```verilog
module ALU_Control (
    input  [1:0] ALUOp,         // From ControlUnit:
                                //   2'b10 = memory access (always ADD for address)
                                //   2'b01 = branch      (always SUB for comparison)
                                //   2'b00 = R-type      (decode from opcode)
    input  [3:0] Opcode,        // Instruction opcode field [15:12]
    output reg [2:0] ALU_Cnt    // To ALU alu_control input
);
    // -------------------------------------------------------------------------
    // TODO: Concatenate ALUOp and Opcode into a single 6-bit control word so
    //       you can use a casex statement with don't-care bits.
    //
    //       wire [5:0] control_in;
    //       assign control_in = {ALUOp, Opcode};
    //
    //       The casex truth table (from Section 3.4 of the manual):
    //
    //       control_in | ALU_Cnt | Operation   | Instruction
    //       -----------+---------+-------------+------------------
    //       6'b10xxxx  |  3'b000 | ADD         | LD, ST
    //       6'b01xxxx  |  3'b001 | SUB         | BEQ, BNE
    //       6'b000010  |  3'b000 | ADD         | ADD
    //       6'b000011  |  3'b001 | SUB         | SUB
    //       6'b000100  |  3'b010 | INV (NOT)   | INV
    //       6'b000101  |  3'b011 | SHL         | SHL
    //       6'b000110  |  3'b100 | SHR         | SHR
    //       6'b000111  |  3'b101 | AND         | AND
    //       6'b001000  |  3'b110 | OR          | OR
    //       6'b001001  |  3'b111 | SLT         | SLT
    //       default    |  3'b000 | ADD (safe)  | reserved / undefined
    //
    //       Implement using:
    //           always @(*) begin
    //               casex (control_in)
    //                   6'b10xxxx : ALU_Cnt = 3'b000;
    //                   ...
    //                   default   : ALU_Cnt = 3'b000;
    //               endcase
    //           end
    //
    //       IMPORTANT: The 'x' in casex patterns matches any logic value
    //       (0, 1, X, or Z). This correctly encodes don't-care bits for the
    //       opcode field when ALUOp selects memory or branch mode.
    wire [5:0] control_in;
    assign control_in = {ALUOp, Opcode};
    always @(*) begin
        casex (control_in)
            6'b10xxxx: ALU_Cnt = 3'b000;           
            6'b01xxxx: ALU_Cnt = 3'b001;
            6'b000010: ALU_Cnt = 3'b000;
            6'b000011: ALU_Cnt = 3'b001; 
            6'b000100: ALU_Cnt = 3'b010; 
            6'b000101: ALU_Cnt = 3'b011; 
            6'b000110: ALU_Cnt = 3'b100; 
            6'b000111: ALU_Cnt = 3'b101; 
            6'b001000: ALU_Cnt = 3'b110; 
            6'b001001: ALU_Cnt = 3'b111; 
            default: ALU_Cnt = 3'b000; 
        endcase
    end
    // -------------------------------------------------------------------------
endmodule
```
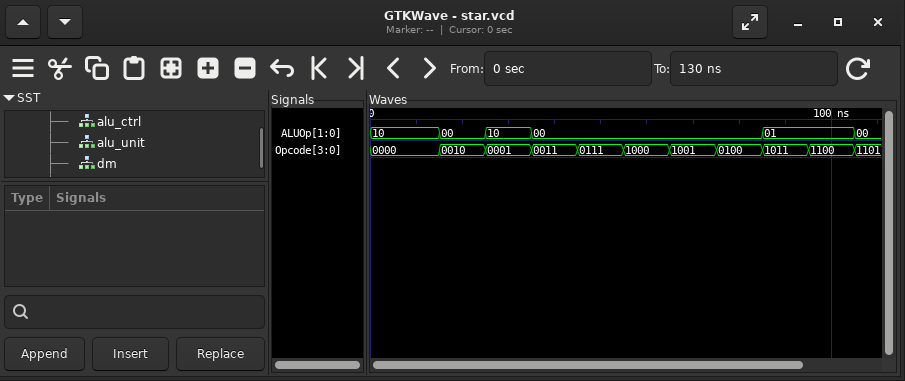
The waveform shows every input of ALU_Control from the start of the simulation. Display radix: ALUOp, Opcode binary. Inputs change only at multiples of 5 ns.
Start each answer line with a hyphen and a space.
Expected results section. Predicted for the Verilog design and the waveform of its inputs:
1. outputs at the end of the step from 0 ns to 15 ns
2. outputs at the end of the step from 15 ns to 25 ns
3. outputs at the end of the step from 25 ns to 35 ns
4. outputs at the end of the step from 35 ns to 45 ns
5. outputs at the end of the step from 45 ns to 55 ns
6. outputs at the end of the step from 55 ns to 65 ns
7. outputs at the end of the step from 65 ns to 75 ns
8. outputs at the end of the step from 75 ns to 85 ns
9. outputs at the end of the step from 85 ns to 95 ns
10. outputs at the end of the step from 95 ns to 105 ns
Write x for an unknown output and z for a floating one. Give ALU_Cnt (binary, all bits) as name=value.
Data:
- ALU_Cnt=000
- ALU_Cnt=000
- ALU_Cnt=000
- ALU_Cnt=001
- ALU_Cnt=101
- ALU_Cnt=110
- ALU_Cnt=111
- ALU_Cnt=010
- ALU_Cnt=001
- ALU_Cnt=001
